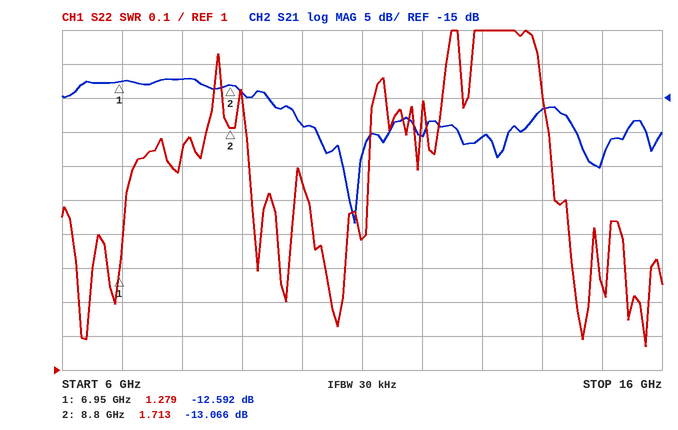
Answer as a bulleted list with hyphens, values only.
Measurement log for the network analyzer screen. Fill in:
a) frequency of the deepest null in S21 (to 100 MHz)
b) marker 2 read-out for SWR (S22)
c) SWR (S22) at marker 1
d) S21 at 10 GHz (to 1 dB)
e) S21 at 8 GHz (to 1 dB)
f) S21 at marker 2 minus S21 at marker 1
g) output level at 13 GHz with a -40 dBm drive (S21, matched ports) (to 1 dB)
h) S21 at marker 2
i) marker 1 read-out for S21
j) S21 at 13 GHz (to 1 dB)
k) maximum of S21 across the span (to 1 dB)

- 10.9 GHz
- 1.713
- 1.279
- -19 dB
- -12 dB
- -0.474 dB
- -61 dBm
- -13.066 dB
- -12.592 dB
- -21 dB
- -12 dB
